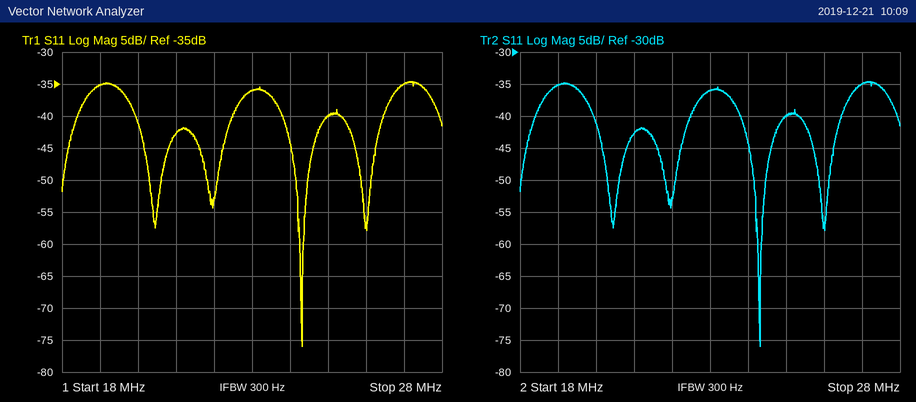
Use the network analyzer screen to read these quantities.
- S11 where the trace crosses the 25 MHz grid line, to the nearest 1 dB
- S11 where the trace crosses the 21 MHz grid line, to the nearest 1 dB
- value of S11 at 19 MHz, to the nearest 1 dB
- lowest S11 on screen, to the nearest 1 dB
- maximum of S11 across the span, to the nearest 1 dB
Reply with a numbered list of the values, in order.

1. -40 dB
2. -43 dB
3. -35 dB
4. -76 dB
5. -35 dB
